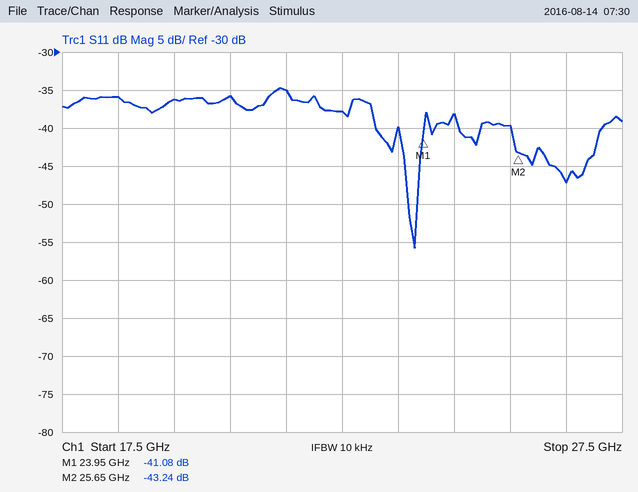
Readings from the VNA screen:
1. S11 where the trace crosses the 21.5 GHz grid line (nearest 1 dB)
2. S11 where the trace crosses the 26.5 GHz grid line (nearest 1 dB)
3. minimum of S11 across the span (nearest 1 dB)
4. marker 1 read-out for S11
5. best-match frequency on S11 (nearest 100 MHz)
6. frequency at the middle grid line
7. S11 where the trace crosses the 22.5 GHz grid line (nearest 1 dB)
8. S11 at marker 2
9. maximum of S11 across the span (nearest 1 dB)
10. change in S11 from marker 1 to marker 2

-35 dB
-47 dB
-56 dB
-41.08 dB
23.8 GHz
22.5 GHz
-38 dB
-43.24 dB
-35 dB
-2.16 dB
